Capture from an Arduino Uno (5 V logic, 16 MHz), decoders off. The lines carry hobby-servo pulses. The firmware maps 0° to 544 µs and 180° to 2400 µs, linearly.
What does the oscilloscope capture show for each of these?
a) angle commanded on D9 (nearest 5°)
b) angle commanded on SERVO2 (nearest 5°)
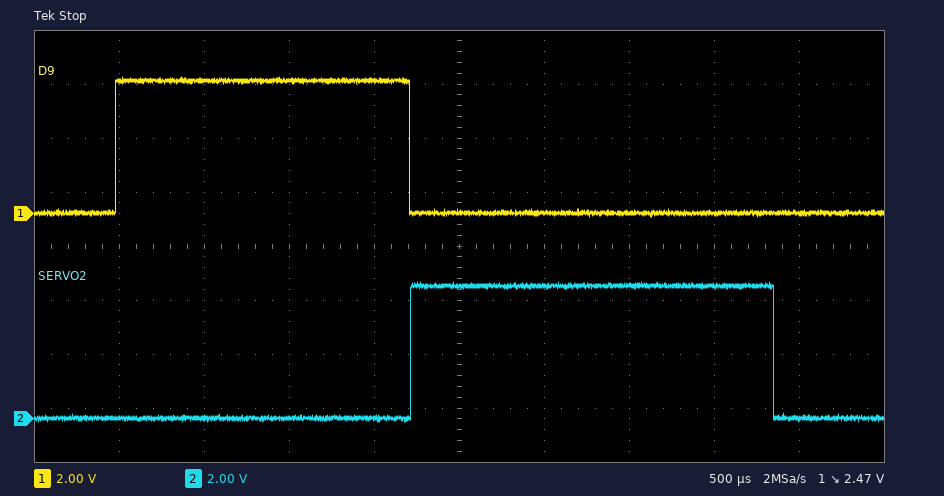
115°
155°
